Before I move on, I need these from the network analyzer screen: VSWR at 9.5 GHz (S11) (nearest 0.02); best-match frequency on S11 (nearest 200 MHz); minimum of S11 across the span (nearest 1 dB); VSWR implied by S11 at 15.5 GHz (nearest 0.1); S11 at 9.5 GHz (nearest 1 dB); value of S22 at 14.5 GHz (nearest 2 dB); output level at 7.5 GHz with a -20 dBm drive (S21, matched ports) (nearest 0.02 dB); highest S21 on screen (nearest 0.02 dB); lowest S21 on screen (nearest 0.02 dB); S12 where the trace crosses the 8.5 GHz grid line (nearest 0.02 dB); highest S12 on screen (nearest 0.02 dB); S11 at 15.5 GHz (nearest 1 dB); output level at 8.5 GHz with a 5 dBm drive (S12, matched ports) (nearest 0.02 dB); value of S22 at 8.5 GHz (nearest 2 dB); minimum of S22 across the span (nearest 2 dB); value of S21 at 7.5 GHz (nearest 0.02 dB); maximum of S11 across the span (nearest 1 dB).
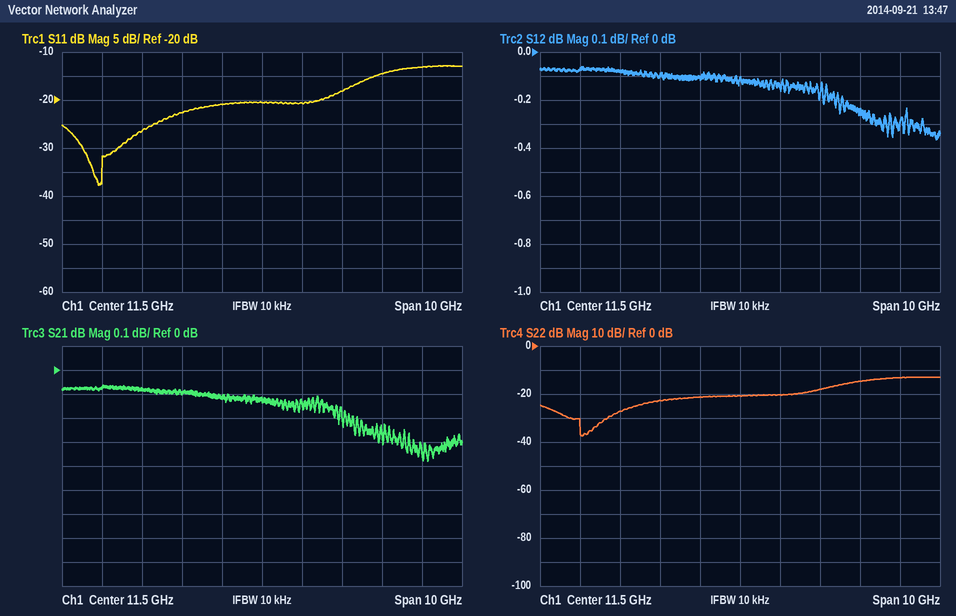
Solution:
1.16
7.4 GHz
-38 dB
1.6
-23 dB
-14 dB
-20.08 dBm
-0.06 dB
-0.38 dB
-0.08 dB
-0.06 dB
-13 dB
4.92 dBm
-28 dB
-38 dB
-0.08 dB
-13 dB
